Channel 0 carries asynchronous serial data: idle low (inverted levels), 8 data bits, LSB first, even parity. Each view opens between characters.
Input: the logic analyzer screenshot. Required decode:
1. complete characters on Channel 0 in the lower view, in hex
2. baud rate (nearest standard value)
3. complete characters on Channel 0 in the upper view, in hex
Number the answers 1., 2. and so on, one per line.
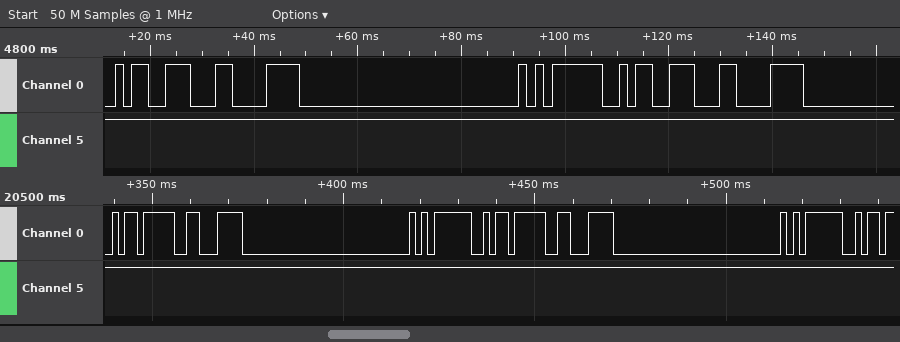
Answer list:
1. 09, 0E, 05, 09, 0E, 05
2. 600 baud
3. 19, 1E, 05, 19, 1E
